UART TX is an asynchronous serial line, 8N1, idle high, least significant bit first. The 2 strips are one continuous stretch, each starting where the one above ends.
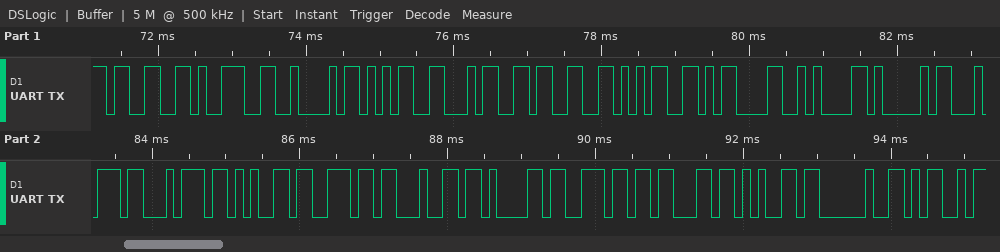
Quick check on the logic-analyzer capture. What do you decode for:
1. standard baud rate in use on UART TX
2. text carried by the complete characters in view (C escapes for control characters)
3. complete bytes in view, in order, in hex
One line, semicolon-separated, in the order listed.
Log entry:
9600 baud; "39B5435\r\nAttendance M"; 33 39 42 35 34 33 35 0D 0A 41 74 74 65 6E 64 61 6E 63 65 20 4D
